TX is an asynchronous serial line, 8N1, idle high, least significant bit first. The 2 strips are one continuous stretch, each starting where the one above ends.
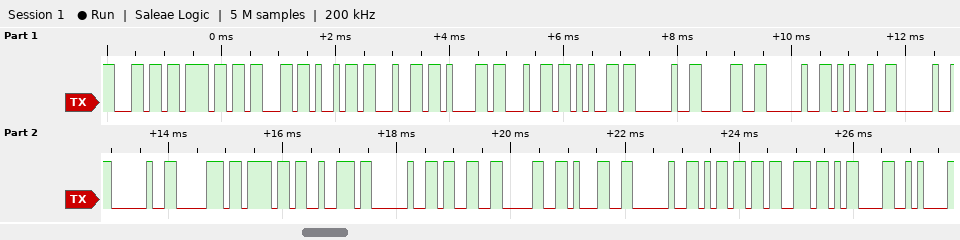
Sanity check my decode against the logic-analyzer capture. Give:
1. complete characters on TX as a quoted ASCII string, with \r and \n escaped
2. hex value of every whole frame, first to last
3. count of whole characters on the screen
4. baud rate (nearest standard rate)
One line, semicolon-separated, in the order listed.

"locidade 0 %  por 301 ms\r\n"; 6C 6F 63 69 64 61 64 65 20 30 20 25 20 20 70 6F 72 20 33 30 31 20 6D 73 0D 0A; 26; 9600 baud
